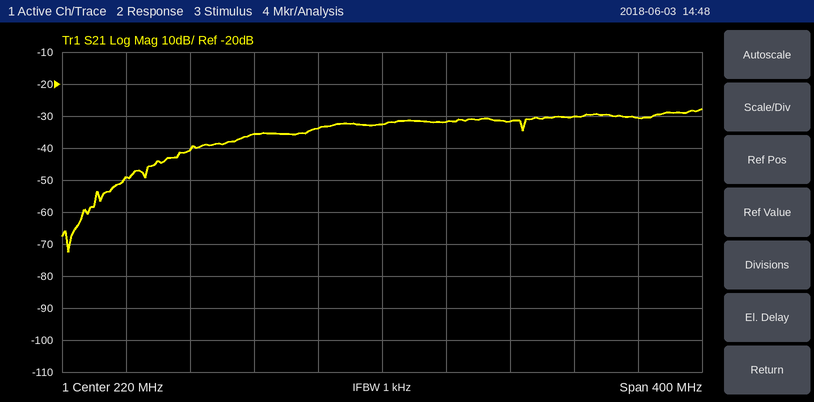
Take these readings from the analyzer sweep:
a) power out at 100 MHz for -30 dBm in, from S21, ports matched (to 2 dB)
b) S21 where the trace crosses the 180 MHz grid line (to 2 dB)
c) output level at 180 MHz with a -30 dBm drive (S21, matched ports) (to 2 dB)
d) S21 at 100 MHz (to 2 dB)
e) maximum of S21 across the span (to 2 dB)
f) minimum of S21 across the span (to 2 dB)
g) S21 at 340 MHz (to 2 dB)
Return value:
-70 dBm
-34 dB
-64 dBm
-40 dB
-28 dB
-72 dB
-30 dB
